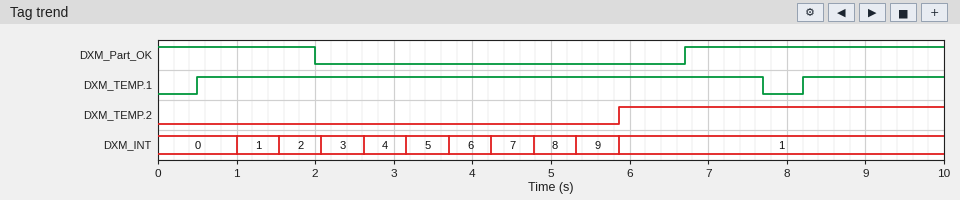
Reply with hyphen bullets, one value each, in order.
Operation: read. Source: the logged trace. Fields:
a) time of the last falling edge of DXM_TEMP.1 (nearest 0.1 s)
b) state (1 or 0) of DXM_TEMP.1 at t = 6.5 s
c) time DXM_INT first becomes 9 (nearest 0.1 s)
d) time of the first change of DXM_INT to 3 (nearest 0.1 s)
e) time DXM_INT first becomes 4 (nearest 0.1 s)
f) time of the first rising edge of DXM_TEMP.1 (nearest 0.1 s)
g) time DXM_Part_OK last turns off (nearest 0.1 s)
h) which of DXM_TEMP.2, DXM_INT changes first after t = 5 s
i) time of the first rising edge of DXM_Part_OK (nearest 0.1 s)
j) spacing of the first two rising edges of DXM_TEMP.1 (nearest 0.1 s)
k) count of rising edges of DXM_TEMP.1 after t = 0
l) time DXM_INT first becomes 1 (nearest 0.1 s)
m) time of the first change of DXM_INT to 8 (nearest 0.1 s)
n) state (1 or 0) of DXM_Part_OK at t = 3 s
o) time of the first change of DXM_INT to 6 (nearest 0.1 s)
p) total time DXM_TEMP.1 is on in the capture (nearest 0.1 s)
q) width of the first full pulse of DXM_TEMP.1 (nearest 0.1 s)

- 7.7 s
- 1
- 5.3 s
- 2.1 s
- 2.6 s
- 0.5 s
- 2.0 s
- DXM_INT
- 6.7 s
- 7.7 s
- 2
- 1.0 s
- 4.8 s
- 0
- 3.7 s
- 9.0 s
- 7.2 s
